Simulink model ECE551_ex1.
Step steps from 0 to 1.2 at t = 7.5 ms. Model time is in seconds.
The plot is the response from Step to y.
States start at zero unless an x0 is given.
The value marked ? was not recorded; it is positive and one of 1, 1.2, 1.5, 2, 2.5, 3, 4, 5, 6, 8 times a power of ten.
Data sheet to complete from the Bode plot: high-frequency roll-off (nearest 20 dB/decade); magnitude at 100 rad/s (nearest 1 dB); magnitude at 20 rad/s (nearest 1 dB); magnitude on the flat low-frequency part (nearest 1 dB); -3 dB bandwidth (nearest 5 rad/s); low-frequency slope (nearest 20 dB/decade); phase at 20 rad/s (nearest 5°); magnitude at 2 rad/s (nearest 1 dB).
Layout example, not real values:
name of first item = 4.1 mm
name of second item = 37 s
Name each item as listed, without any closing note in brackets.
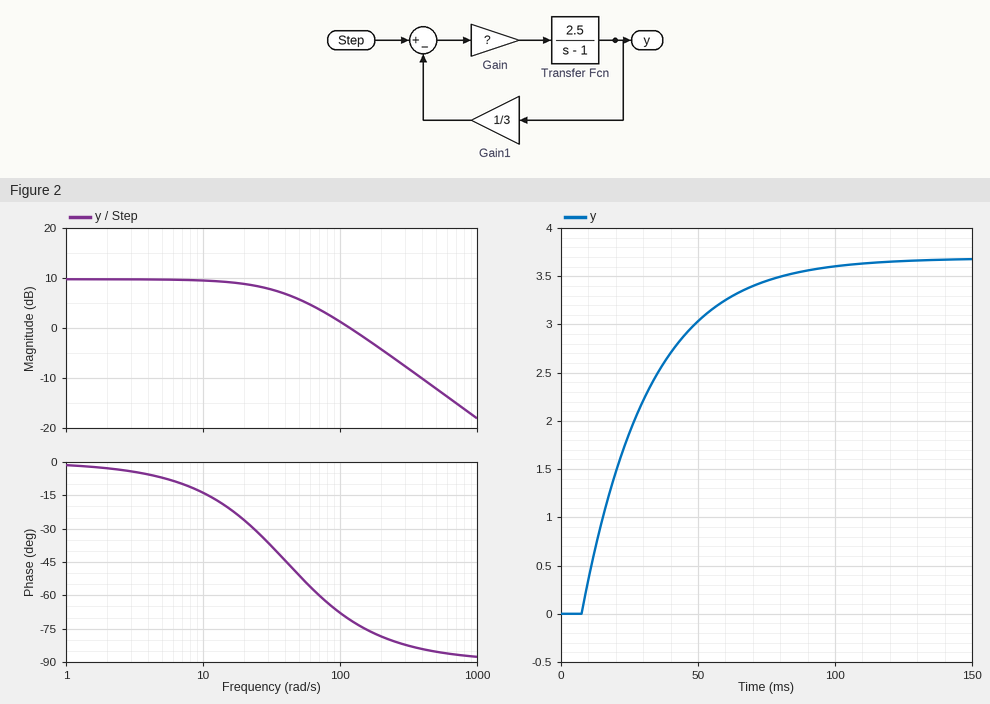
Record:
high-frequency roll-off = -20 dB/decade
magnitude at 100 rad/s = 1 dB
magnitude at 20 rad/s = 9 dB
magnitude on the flat low-frequency part = 10 dB
-3 dB bandwidth = 40 rad/s
low-frequency slope = 0 dB/decade
phase at 20 rad/s = -25°
magnitude at 2 rad/s = 10 dB
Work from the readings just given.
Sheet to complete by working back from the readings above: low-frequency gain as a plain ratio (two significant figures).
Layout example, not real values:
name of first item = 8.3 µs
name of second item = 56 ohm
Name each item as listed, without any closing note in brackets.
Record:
low-frequency gain as a plain ratio = 3.2
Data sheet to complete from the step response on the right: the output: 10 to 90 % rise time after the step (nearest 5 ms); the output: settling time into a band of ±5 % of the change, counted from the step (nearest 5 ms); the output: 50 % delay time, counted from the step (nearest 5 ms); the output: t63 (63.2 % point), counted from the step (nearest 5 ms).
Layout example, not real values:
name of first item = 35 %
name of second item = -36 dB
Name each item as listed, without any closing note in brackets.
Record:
the output: 10 to 90 % rise time after the step = 55 ms
the output: settling time into a band of ±5 % of the change, counted from the step = 75 ms
the output: 50 % delay time, counted from the step = 15 ms
the output: t63 (63.2 % point), counted from the step = 25 ms
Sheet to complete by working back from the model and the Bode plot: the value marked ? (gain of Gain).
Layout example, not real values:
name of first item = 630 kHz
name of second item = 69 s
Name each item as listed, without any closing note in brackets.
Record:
the value marked ? = 50
